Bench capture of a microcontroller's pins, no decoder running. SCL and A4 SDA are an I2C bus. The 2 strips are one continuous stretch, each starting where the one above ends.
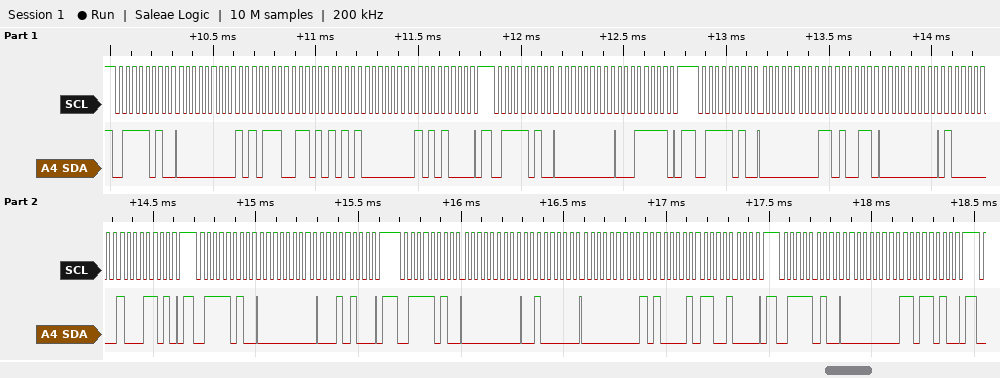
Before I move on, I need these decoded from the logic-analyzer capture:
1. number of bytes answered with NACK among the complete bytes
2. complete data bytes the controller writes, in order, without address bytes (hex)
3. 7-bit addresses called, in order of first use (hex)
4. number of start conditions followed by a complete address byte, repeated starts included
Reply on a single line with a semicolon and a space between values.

0; 00 AE D5 80 A8 00 1F 00 D3 00 40 8D 00 14 00 20 00 A1 C8 00 DA; 0x3D; 6
